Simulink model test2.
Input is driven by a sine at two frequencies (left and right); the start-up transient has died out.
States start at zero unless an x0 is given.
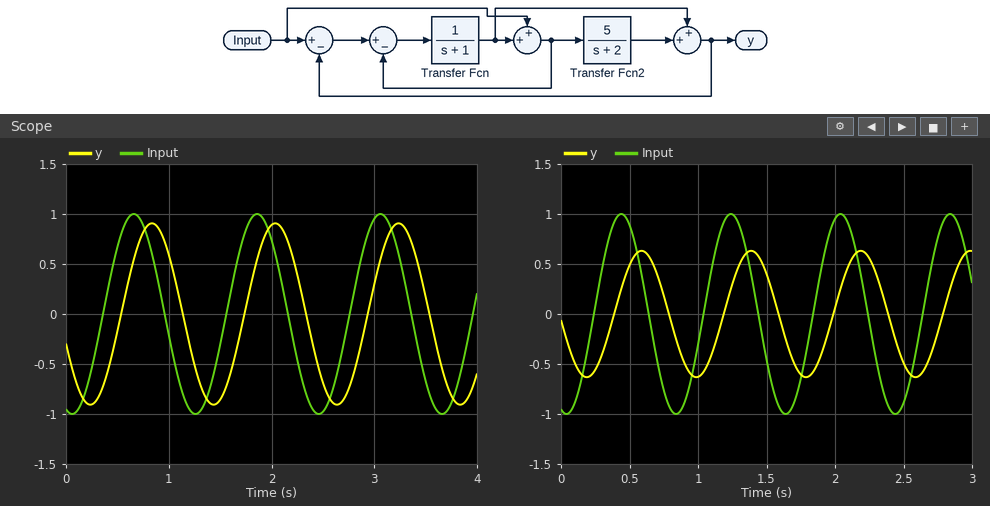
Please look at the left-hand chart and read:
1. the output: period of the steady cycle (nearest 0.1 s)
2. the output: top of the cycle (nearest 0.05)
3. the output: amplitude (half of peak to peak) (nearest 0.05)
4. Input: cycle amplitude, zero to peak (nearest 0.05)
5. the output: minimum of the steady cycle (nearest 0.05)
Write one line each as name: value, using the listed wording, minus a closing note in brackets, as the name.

the output: period of the steady cycle: 1.2 s
the output: top of the cycle: 0.90
the output: amplitude (half of peak to peak): 0.90
Input: cycle amplitude, zero to peak: 1.00
the output: minimum of the steady cycle: -0.90
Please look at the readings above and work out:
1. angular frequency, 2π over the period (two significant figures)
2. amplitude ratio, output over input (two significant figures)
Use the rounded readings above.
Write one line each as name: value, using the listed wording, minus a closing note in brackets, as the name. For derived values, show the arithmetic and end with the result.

angular frequency, 2π over the period: 2π / 1.2 = 5.2 rad/s
amplitude ratio, output over input: 0.9 / 1 = 0.90
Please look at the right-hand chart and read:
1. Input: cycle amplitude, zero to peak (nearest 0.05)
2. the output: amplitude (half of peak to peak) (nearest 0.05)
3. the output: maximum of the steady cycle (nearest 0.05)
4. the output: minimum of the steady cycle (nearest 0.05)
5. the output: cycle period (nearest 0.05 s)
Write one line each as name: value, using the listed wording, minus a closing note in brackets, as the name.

Input: cycle amplitude, zero to peak: 1.00
the output: amplitude (half of peak to peak): 0.65
the output: maximum of the steady cycle: 0.65
the output: minimum of the steady cycle: -0.65
the output: cycle period: 0.80 s
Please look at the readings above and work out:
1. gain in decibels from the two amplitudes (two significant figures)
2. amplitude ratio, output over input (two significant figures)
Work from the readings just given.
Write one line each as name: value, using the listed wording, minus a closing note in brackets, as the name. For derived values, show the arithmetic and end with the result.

gain in decibels from the two amplitudes: 20 log10(0.65 / 1) = -3.7 dB
amplitude ratio, output over input: 0.65 / 1 = 0.65
